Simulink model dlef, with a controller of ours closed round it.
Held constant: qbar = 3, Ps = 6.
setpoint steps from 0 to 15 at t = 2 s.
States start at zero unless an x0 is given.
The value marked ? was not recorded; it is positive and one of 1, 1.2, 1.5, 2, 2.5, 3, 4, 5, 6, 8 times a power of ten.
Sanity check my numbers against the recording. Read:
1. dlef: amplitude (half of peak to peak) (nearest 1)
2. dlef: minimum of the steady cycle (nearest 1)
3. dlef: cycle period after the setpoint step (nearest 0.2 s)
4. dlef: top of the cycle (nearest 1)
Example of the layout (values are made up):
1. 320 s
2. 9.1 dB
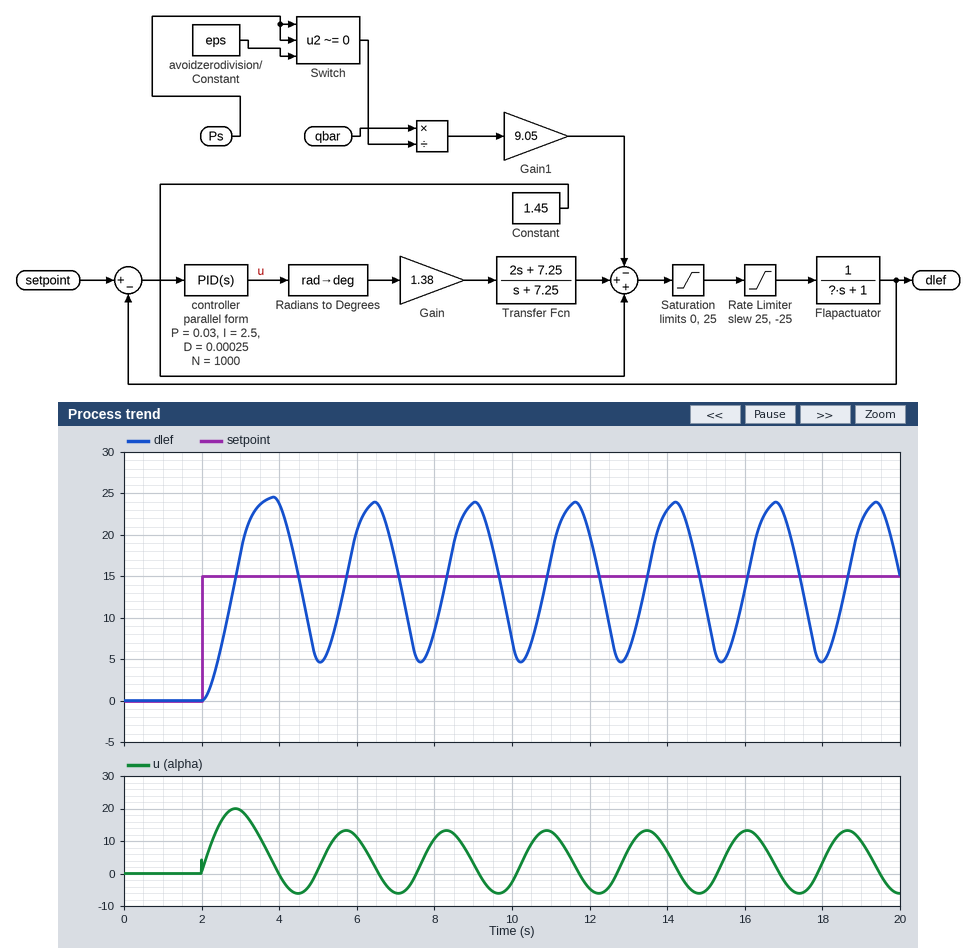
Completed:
1. 10
2. 5
3. 2.6 s
4. 24
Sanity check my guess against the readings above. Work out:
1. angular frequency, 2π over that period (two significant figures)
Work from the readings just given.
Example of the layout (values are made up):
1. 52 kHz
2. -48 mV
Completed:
1. 2.4 rad/s
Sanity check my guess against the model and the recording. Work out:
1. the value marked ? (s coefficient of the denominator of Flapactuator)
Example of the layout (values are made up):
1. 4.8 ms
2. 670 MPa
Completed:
1. 0.3
